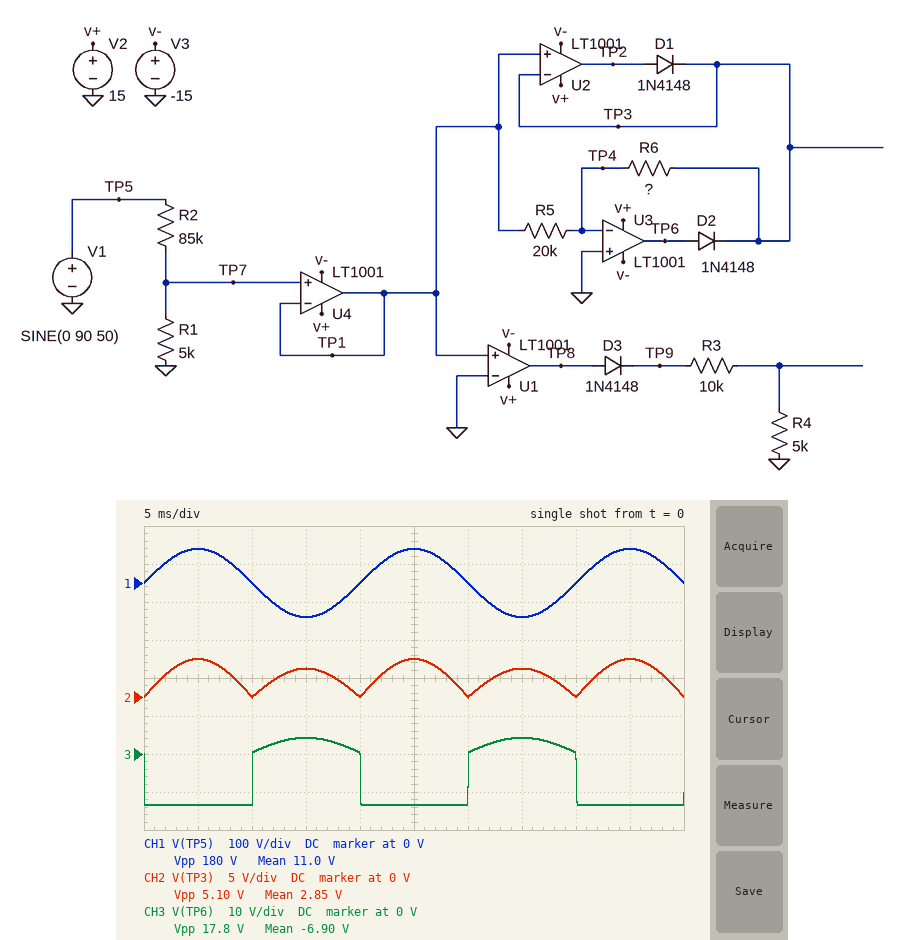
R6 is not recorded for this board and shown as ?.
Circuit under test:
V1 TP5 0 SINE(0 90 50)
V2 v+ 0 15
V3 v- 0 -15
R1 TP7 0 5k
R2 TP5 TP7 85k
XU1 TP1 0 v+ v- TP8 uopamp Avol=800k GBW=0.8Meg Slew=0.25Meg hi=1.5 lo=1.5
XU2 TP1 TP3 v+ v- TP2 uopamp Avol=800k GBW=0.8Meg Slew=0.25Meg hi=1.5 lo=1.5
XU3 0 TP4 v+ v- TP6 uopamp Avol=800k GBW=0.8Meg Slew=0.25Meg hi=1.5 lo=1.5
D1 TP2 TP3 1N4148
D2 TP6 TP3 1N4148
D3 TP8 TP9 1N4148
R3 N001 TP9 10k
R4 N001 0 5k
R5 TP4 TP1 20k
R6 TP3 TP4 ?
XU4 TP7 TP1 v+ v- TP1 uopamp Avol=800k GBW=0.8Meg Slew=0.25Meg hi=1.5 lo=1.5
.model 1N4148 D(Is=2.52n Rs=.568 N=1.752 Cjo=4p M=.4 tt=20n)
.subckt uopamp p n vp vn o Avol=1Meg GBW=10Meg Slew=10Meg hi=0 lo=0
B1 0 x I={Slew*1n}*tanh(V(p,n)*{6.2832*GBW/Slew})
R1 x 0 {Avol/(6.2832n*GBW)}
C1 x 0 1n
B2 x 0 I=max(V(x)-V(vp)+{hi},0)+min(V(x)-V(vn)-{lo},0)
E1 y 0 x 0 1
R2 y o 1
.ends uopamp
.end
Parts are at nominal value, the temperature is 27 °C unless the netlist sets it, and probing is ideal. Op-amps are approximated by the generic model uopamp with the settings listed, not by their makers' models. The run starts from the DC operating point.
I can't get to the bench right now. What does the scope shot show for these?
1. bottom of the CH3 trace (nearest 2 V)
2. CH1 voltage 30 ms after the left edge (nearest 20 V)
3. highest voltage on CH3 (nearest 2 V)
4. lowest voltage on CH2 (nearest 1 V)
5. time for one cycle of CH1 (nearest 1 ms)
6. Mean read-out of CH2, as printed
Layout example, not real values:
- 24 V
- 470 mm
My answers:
- -14 V
- 0 V
- 4 V
- 0 V
- 20 ms
- 2.85 V
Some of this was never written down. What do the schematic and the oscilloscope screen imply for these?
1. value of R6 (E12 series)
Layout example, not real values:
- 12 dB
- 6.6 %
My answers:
- 15 kΩ
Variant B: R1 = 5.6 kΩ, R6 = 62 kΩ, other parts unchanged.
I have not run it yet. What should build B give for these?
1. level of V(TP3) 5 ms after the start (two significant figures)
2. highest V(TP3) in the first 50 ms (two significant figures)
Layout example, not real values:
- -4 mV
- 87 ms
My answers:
- 5.6 V
- 13 V
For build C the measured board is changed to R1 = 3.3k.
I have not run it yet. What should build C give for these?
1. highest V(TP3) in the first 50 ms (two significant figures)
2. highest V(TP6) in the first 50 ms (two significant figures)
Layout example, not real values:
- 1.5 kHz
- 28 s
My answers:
- 3.4 V
- 3.0 V
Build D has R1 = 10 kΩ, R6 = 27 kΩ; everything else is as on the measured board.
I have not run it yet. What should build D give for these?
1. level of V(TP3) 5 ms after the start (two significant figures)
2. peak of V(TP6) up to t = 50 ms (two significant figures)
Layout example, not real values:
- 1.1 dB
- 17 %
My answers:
- 9.5 V
- 13 V
